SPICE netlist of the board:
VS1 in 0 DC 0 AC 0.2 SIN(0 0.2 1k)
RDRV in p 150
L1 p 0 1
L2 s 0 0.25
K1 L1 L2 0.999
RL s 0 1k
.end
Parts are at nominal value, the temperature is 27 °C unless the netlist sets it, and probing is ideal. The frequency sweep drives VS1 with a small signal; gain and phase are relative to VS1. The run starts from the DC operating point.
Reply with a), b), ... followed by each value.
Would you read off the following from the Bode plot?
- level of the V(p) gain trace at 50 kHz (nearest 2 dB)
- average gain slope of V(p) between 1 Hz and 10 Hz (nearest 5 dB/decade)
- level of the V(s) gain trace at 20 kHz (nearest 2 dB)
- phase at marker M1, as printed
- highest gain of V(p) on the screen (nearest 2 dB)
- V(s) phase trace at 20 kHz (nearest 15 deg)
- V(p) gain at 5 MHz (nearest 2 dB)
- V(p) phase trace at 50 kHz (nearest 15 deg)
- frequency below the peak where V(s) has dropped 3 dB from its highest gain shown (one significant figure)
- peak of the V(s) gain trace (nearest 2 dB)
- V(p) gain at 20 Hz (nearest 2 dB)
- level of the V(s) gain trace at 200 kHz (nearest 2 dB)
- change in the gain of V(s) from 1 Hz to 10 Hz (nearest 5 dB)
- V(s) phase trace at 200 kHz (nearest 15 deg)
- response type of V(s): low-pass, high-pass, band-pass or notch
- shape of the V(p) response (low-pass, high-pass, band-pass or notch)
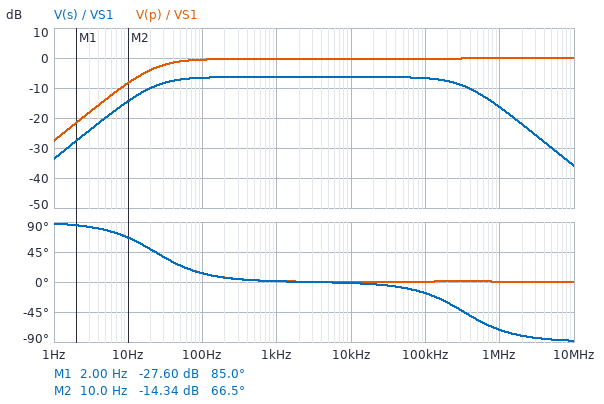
a) 0 dB
b) 20 dB/decade
c) -6 dB
d) 85.0 deg
e) 0 dB
f) 0 deg
g) 0 dB
h) 0 deg
i) 20 Hz
j) -6 dB
k) -4 dB
l) -8 dB
m) 20 dB
n) -30 deg
o) band-pass
p) high-pass
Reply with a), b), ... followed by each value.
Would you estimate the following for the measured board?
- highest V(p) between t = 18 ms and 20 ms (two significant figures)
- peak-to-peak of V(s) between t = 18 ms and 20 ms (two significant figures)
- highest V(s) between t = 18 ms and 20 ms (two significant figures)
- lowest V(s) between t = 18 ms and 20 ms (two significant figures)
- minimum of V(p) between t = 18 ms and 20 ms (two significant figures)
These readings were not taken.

a) 190 mV
b) 190 mV
c) 96 mV
d) -96 mV
e) -190 mV
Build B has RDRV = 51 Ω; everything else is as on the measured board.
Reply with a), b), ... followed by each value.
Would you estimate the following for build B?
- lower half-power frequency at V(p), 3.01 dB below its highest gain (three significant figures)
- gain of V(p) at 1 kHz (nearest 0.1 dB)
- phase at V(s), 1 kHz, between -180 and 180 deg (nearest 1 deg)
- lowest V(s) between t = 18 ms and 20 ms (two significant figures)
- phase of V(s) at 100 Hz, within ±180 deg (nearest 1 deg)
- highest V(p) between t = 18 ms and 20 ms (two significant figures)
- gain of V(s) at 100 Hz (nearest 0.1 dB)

a) 8.22 Hz
b) -0.1 dB
c) 0 deg
d) -99 mV
e) 5 deg
f) 200 mV
g) -6.2 dB
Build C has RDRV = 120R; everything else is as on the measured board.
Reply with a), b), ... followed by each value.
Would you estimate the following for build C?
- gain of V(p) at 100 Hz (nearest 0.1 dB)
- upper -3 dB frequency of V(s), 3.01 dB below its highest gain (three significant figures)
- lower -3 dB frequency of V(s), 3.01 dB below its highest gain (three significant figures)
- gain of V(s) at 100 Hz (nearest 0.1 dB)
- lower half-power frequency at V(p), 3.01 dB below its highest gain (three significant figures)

a) -0.4 dB
b) 328 kHz
c) 18.5 Hz
d) -6.4 dB
e) 19.7 Hz
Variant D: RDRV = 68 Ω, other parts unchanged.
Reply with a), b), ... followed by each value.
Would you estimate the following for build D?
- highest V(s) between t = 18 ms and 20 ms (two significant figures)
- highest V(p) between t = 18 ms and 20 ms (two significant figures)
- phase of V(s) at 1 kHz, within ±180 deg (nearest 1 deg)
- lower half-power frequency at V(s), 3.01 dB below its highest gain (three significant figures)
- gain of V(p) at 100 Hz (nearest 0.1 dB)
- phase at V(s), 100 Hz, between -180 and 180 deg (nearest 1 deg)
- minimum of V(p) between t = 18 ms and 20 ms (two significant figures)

a) 98 mV
b) 200 mV
c) 0 deg
d) 10.6 Hz
e) -0.2 dB
f) 6 deg
g) -200 mV
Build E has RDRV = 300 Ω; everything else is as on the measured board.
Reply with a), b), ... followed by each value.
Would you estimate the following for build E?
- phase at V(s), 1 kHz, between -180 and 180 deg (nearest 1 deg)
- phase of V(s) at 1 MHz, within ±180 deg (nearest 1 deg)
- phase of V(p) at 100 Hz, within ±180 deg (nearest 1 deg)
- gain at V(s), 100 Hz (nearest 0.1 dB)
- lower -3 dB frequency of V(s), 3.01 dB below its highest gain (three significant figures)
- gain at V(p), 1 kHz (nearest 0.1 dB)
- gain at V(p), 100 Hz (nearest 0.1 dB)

a) 2 deg
b) -71 deg
c) 24 deg
d) -7.4 dB
e) 44.4 Hz
f) -0.6 dB
g) -1.4 dB
